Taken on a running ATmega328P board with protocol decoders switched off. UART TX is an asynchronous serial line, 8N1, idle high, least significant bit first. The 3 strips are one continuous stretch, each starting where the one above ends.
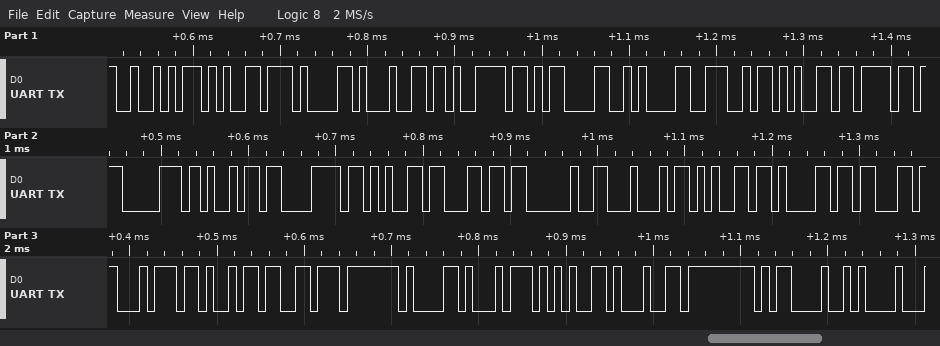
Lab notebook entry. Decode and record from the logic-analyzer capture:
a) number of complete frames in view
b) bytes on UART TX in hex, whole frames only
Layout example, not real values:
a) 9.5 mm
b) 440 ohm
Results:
a) 29
b) 52 65 61 64 79 0D 0A 4E 65 6F 70 69 78 65 6C 20 44 65 61 63 74 69 76 61 74 65 64 0D 0A
